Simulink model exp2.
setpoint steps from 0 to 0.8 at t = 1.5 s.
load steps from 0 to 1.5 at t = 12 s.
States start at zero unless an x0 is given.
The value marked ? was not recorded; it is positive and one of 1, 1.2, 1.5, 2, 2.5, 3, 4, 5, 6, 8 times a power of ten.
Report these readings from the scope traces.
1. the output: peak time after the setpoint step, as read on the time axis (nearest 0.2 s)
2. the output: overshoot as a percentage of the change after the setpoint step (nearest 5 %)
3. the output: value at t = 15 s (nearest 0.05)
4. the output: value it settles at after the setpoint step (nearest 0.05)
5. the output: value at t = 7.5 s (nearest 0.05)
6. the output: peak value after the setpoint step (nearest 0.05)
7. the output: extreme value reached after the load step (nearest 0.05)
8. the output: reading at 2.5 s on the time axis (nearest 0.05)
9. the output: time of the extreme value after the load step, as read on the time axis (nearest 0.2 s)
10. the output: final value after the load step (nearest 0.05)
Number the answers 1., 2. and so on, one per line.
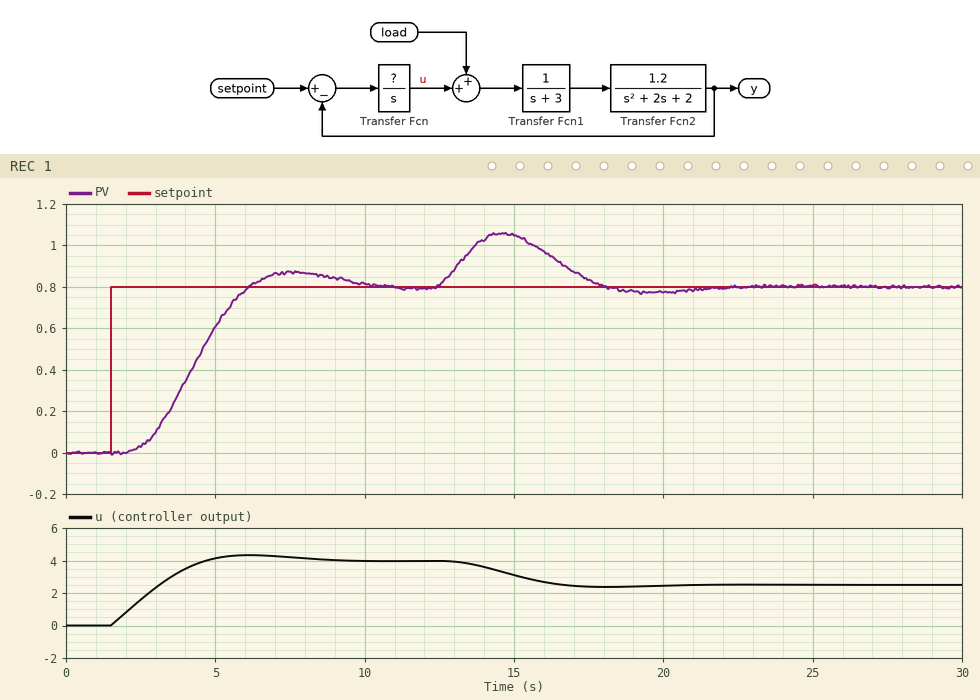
1. 7.6 s
2. 10 %
3. 1.05
4. 0.80
5. 0.85
6. 0.85
7. 1.05
8. 0.05
9. 14.6 s
10. 0.80
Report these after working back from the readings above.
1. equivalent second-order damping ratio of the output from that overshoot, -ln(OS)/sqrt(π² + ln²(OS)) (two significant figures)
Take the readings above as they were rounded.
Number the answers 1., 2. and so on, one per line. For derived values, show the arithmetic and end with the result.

1. ln(0.1) = -2.303; 2.303 / sqrt(9.870 + 5.302) = 0.59
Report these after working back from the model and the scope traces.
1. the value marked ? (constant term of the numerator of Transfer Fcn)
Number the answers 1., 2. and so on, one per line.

1. 2
